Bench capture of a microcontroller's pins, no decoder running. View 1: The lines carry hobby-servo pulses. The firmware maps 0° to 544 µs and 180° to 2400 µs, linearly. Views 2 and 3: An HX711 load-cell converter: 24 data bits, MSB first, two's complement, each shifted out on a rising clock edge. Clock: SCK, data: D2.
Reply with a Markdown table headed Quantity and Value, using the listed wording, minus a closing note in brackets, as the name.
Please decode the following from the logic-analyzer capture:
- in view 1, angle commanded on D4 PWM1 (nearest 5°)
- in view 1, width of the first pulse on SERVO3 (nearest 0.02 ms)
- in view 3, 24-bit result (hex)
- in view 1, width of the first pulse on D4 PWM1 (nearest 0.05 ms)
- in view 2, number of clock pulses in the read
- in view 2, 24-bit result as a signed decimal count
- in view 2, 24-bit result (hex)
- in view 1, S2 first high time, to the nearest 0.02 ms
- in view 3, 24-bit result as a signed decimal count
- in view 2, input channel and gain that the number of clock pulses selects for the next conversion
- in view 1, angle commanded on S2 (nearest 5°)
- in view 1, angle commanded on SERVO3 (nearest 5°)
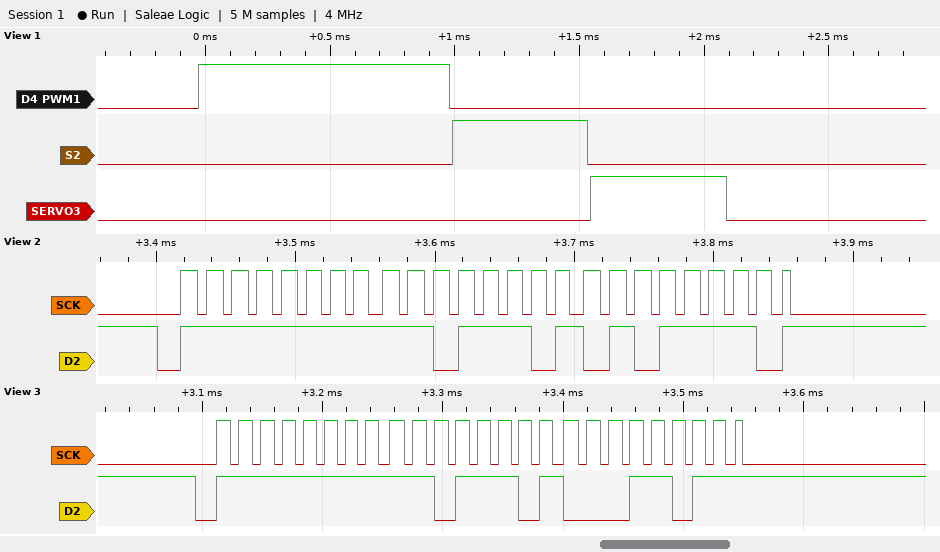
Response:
| Quantity | Value |
|---|---|
| in view 1, angle commanded on D4 PWM1 | 45° |
| in view 1, width of the first pulse on SERVO3 | 0.54 ms |
| in view 3, 24-bit result | 0xFFDD1B |
| in view 1, width of the first pulse on D4 PWM1 | 1.00 ms |
| in view 2, number of clock pulses in the read | 25 |
| in view 2, 24-bit result as a signed decimal count | -8866 |
| in view 2, 24-bit result | 0xFFDD5E |
| in view 1, S2 first high time, to the nearest 0.02 ms | 0.54 ms |
| in view 3, 24-bit result as a signed decimal count | -8933 |
| in view 2, input channel and gain that the number of clock pulses selects for the next conversion | channel A, gain 128 |
| in view 1, angle commanded on S2 | 0° |
| in view 1, angle commanded on SERVO3 | 0° |
